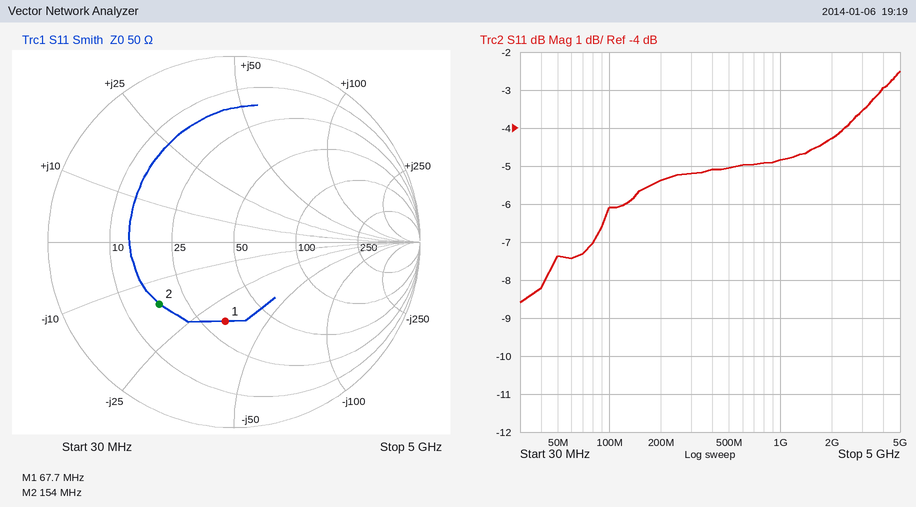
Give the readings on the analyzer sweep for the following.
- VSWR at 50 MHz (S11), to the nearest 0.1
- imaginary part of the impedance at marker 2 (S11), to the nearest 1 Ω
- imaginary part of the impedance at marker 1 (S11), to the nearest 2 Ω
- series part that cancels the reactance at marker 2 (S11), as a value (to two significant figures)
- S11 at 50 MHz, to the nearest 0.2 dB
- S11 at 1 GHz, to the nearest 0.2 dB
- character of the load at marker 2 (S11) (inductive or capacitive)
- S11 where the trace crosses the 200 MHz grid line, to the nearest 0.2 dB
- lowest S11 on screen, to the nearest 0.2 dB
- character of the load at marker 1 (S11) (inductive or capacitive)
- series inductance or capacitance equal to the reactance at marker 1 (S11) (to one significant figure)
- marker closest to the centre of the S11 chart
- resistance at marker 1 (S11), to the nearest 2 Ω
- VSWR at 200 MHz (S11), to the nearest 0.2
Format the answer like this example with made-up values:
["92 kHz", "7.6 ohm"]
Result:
["2.5", "-16 Ω", "-34 Ω", "17 nH", "-7.4 dB", "-4.8 dB", "capacitive", "-5.4 dB", "-8.6 dB", "capacitive", "70 pF", "marker 1", "32 Ω", "3.4"]
